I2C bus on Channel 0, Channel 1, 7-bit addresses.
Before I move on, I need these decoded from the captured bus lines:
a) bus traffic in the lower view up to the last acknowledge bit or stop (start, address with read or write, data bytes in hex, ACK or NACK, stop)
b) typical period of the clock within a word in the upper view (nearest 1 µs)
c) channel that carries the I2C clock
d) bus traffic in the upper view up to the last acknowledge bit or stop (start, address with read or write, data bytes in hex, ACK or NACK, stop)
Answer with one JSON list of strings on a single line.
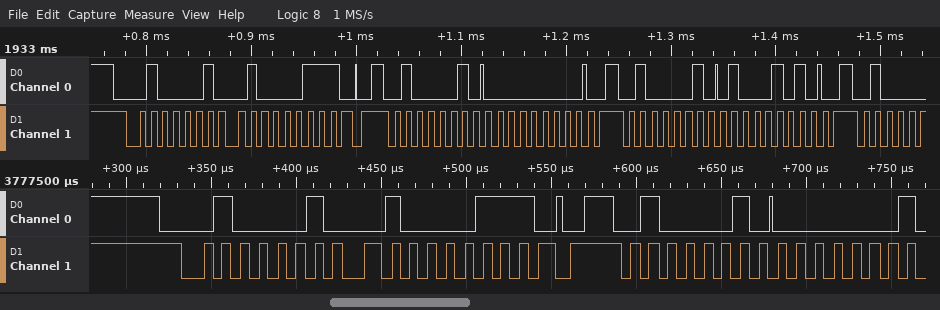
["start, address 21 write ACK, 87 ACK, stop, start, address 21 write ACK", "11 µs", "Channel 1", "start, address 21 write ACK, 87 ACK, stop, start, address 21 write ACK, 00 ACK, stop, start, address 21 write ACK, 8A ACK, stop"]
